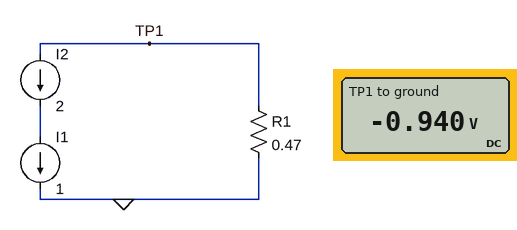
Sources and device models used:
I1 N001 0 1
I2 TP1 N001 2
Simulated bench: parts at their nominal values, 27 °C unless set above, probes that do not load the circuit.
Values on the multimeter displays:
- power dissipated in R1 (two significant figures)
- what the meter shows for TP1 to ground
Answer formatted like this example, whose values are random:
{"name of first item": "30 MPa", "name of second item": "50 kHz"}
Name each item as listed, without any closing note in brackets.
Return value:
{"power dissipated in R1": "1.9 W", "what the meter shows for TP1 to ground": "-0.940 V"}
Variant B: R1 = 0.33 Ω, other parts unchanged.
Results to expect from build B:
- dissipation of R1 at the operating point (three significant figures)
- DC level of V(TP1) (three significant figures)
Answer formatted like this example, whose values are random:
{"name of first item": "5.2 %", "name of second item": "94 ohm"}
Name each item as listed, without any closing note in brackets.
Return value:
{"dissipation of R1 at the operating point": "1.32 W", "DC level of V(TP1)": "-660 mV"}
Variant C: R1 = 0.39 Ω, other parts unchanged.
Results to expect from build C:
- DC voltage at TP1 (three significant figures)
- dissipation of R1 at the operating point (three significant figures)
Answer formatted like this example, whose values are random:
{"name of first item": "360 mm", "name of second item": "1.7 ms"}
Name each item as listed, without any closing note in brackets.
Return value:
{"DC voltage at TP1": "-780 mV", "dissipation of R1 at the operating point": "1.56 W"}
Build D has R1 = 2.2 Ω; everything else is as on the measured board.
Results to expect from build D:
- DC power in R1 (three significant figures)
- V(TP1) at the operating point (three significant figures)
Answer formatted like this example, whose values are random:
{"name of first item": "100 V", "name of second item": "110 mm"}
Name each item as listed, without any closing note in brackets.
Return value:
{"DC power in R1": "8.80 W", "V(TP1) at the operating point": "-4.40 V"}
